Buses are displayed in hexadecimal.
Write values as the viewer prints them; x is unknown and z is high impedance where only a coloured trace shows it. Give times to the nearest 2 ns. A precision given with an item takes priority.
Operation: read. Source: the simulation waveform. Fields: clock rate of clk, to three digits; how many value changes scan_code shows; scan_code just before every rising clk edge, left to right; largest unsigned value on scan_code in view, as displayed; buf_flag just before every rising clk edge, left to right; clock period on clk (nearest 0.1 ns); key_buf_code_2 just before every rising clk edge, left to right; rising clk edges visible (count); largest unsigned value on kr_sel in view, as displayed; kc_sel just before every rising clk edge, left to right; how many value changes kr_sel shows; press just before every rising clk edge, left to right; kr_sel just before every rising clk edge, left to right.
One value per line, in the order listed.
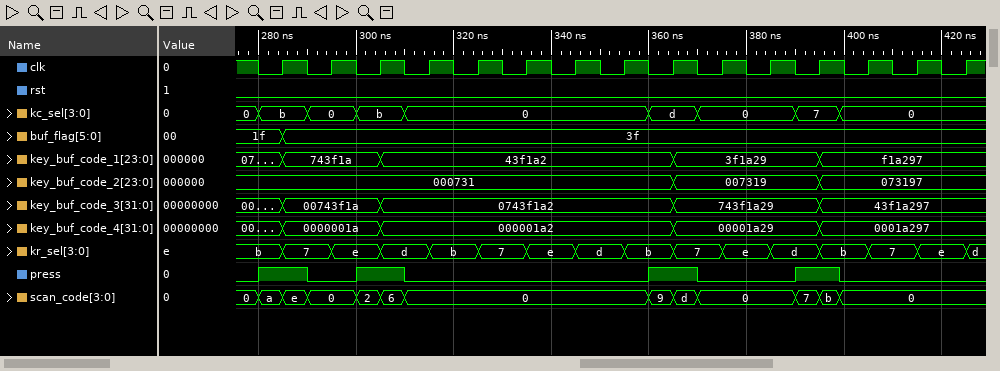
100 MHz
12
a, 0, 2, 0, 0, 0, 0, 0, 9, 0, 0, 7, 0, 0, 0
e
1f, 3f, 3f, 3f, 3f, 3f, 3f, 3f, 3f, 3f, 3f, 3f, 3f, 3f, 3f
10 ns
000731, 000731, 000731, 000731, 000731, 000731, 000731, 000731, 000731, 007319, 007319, 007319, 073197, 073197, 073197
15
e
b, 0, b, 0, 0, 0, 0, 0, d, 0, 0, 7, 0, 0, 0
15
1 0 1 0 0 0 0 0 1 0 0 1 0 0 0
b, 7, e, d, b, 7, e, d, b, 7, e, d, b, 7, e
